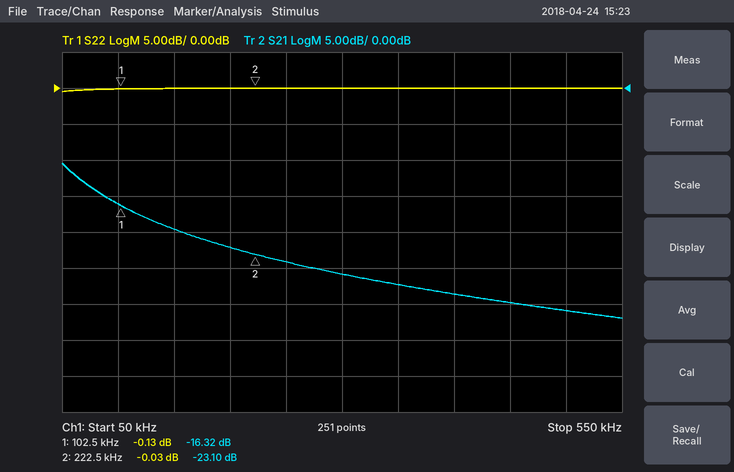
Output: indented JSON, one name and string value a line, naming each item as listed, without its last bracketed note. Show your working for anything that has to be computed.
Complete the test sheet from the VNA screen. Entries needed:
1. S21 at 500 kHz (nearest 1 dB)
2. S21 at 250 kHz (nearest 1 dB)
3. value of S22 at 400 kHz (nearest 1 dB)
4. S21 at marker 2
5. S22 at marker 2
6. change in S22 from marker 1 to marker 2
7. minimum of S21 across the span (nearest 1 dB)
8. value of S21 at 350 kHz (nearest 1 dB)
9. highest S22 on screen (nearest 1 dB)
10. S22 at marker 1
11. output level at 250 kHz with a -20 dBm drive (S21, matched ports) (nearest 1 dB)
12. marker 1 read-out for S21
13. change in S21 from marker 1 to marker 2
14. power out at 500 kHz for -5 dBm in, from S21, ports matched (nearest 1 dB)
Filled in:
{
  "S21 at 500 kHz": "-31 dB",
  "S21 at 250 kHz": "-24 dB",
  "value of S22 at 400 kHz": "0 dB",
  "S21 at marker 2": "-23.10 dB",
  "S22 at marker 2": "-0.03 dB",
  "change in S22 from marker 1 to marker 2": "-0.03 − (-0.13) = 0.10 dB",
  "minimum of S21 across the span": "-32 dB",
  "value of S21 at 350 kHz": "-27 dB",
  "highest S22 on screen": "0 dB",
  "S22 at marker 1": "-0.13 dB",
  "output level at 250 kHz with a -20 dBm drive (S21, matched ports)": "-20 dBm + (-24 dB) = -44 dBm",
  "marker 1 read-out for S21": "-16.32 dB",
  "change in S21 from marker 1 to marker 2": "-23.1 − (-16.32) = -6.78 dB",
  "power out at 500 kHz for -5 dBm in, from S21, ports matched": "-5 dBm + (-31 dB) = -36 dBm"
}
